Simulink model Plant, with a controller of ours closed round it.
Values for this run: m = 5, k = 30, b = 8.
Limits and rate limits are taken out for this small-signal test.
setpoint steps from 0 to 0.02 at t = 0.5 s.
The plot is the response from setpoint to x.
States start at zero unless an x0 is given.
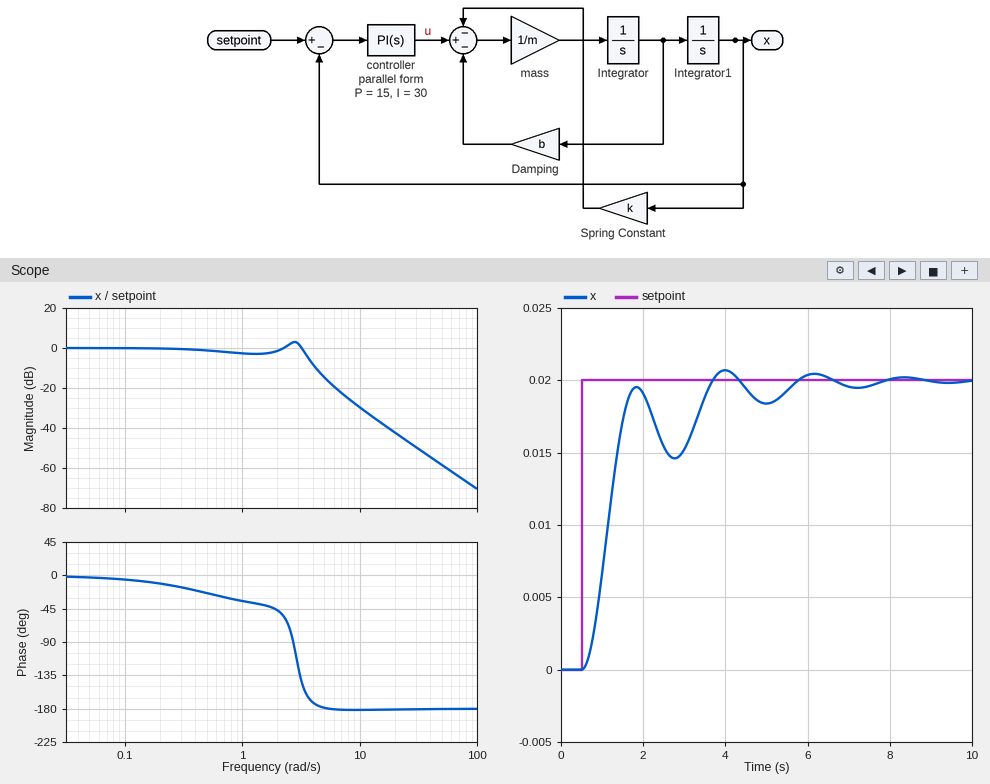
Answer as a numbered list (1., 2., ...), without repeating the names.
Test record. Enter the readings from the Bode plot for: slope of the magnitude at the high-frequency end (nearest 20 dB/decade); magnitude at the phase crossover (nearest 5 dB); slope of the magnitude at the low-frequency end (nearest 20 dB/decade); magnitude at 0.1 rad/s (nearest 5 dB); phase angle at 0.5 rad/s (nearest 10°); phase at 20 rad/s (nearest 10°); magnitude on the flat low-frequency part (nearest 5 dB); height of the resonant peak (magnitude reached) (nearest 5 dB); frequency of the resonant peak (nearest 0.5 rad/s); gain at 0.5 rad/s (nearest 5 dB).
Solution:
1. -40 dB/decade
2. -15 dB
3. 0 dB/decade
4. 0 dB
5. -20°
6. -180°
7. 0 dB
8. 5 dB
9. 3.0 rad/s
10. 0 dB
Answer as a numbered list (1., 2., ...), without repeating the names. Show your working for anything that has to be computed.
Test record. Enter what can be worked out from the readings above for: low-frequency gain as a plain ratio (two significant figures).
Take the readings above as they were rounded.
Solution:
1. 10^(0 / 20) = 1.0
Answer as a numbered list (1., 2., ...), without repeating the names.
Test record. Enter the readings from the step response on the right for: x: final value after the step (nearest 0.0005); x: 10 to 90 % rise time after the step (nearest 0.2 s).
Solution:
1. 0.0200
2. 0.8 s
